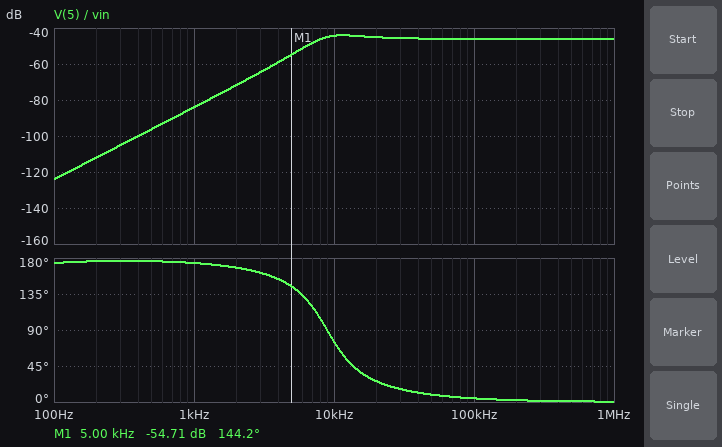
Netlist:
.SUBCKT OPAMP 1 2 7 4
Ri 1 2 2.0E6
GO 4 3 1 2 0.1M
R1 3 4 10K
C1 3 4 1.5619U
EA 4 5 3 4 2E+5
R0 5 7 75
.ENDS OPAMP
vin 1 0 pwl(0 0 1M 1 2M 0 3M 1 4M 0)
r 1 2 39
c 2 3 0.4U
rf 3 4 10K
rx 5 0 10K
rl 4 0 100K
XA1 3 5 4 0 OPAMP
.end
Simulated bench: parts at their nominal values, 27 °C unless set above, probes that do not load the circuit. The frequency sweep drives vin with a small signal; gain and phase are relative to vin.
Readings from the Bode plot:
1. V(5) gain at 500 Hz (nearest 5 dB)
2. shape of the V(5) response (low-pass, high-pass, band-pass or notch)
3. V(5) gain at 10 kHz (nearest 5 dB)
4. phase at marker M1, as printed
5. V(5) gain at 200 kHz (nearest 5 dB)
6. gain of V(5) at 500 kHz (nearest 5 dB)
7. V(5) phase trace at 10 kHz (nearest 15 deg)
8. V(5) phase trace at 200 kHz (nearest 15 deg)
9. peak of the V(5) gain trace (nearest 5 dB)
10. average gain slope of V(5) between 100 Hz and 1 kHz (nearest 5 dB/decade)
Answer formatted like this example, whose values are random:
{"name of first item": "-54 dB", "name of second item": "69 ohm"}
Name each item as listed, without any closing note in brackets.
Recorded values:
{"V(5) gain at 500 Hz": "-95 dB", "shape of the V(5) response": "high-pass", "V(5) gain at 10 kHz": "-45 dB", "phase at marker M1, as printed": "144.2 deg", "V(5) gain at 200 kHz": "-45 dB", "gain of V(5) at 500 kHz": "-45 dB", "V(5) phase trace at 10 kHz": "75 deg", "V(5) phase trace at 200 kHz": "0 deg", "peak of the V(5) gain trace": "-45 dB", "average gain slope of V(5) between 100 Hz and 1 kHz": "40 dB/decade"}
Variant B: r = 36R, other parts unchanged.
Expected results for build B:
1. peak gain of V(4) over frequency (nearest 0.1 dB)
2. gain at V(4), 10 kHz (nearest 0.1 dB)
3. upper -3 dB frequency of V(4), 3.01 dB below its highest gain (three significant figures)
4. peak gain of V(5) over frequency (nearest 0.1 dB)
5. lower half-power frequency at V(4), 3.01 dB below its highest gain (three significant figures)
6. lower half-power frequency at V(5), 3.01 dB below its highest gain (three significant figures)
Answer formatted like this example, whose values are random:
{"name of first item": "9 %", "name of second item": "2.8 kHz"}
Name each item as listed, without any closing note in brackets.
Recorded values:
{"peak gain of V(4) over frequency": "48.8 dB", "gain at V(4), 10 kHz": "48.5 dB", "upper -3 dB frequency of V(4), 3.01 dB below its highest gain": "13.3 kHz", "peak gain of V(5) over frequency": "-43.5 dB", "lower half-power frequency at V(4), 3.01 dB below its highest gain": "6.01 kHz", "lower half-power frequency at V(5), 3.01 dB below its highest gain": "7.51 kHz"}
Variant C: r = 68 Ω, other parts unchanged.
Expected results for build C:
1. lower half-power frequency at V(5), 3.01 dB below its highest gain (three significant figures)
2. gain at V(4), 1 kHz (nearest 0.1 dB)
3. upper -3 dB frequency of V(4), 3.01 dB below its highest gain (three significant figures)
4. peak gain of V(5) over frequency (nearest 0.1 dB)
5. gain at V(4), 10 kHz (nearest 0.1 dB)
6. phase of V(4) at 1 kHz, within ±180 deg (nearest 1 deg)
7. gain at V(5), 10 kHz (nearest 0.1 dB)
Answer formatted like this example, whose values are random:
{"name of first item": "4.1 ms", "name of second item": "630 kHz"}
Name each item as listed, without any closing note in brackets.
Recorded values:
{"lower half-power frequency at V(5), 3.01 dB below its highest gain": "9.70 kHz", "gain at V(4), 1 kHz": "28.0 dB", "upper -3 dB frequency of V(4), 3.01 dB below its highest gain": "18.0 kHz", "peak gain of V(5) over frequency": "-46.1 dB", "gain at V(4), 10 kHz": "43.2 dB", "phase of V(4) at 1 kHz, within ±180 deg": "-100 deg", "gain at V(5), 10 kHz": "-48.9 dB"}
